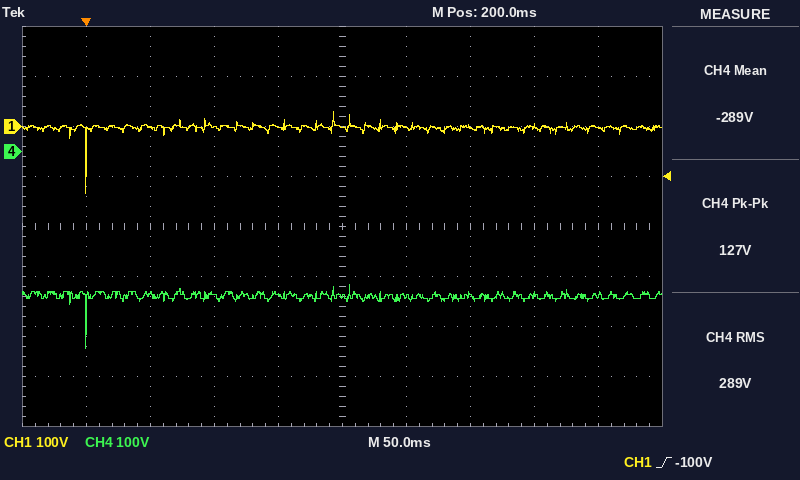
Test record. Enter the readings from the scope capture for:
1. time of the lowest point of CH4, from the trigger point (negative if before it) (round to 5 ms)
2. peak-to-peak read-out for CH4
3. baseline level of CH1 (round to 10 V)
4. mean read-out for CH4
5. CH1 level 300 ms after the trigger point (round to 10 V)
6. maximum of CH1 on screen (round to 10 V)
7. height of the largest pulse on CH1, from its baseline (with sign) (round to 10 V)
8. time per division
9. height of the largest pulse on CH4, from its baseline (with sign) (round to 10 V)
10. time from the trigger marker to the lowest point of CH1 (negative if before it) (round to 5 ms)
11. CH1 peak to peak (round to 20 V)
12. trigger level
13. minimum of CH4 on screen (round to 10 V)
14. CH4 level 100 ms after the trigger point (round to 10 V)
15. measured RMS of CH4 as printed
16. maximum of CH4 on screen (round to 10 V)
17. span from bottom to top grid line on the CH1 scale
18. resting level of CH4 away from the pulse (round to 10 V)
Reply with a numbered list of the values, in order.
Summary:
1. 0 ms
2. 127 V
3. 0 V
4. -289 V
5. 0 V
6. 30 V
7. -130 V
8. 50 ms
9. -100 V
10. 0 ms
11. 160 V
12. -100 V
13. -390 V
14. -290 V
15. 289 V
16. -270 V
17. 800 V
18. -290 V
